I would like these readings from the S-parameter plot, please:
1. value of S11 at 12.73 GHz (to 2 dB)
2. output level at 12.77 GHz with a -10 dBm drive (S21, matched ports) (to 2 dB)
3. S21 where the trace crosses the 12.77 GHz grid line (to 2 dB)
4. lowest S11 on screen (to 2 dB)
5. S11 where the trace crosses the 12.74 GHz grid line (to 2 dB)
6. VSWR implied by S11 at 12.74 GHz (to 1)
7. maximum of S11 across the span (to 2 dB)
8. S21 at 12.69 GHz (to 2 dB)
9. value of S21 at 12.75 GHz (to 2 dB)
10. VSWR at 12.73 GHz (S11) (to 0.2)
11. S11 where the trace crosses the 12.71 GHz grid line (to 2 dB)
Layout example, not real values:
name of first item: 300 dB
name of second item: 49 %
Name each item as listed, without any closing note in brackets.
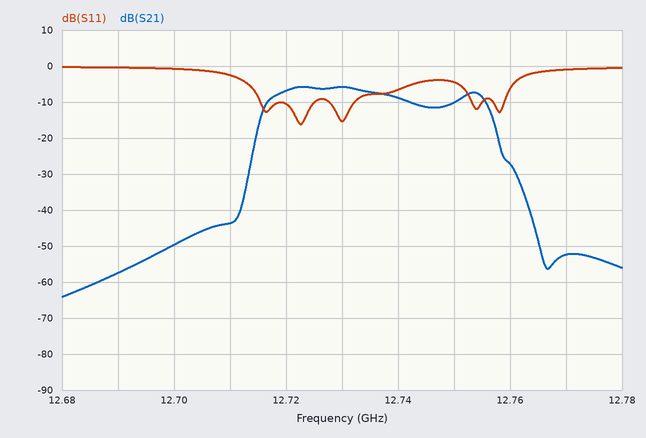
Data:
value of S11 at 12.73 GHz: -16 dB
output level at 12.77 GHz with a -10 dBm drive (S21, matched ports): -62 dBm
S21 where the trace crosses the 12.77 GHz grid line: -52 dB
lowest S11 on screen: -16 dB
S11 where the trace crosses the 12.74 GHz grid line: -6 dB
VSWR implied by S11 at 12.74 GHz: 3
maximum of S11 across the span: 0 dB
S21 at 12.69 GHz: -58 dB
value of S21 at 12.75 GHz: -10 dB
VSWR at 12.73 GHz (S11): 1.4
S11 where the trace crosses the 12.71 GHz grid line: -2 dB
